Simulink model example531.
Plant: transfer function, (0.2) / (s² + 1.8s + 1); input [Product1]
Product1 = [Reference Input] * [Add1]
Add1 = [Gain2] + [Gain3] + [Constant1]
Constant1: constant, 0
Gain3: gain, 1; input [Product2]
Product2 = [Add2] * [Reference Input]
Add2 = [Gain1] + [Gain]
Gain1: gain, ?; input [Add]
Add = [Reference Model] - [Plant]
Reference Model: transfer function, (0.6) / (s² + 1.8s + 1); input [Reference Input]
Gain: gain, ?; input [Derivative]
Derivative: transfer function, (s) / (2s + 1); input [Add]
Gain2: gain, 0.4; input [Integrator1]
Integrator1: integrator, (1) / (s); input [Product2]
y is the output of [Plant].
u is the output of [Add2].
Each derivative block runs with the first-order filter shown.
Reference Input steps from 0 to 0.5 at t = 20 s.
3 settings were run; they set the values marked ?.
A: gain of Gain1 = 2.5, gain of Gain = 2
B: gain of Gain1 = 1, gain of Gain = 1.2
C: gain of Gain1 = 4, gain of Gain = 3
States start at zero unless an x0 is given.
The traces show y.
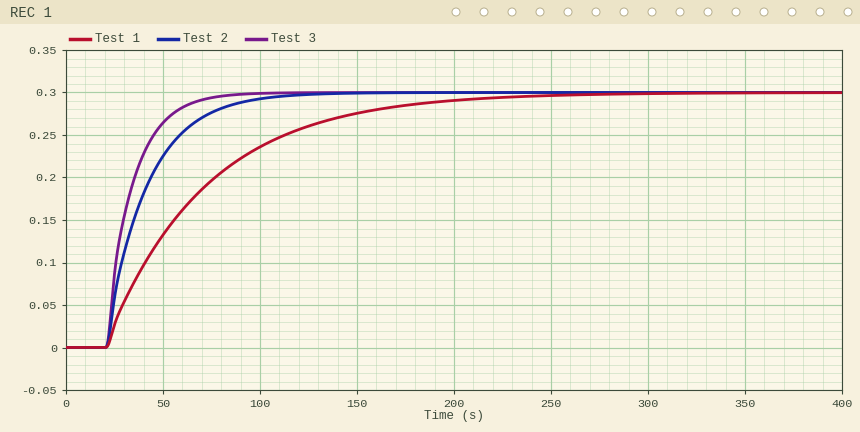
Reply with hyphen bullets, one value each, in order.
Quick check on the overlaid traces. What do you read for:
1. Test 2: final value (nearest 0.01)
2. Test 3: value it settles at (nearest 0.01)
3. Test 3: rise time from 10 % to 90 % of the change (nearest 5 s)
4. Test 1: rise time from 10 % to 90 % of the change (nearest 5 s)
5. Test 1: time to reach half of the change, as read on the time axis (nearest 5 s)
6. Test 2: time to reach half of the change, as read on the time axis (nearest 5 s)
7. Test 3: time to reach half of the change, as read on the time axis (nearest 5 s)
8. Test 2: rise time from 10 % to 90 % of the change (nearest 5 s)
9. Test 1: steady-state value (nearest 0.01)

- 0.30
- 0.30
- 30 s
- 115 s
- 55 s
- 35 s
- 30 s
- 45 s
- 0.30
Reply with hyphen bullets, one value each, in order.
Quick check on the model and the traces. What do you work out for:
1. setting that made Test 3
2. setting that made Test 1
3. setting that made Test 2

- C
- B
- A
